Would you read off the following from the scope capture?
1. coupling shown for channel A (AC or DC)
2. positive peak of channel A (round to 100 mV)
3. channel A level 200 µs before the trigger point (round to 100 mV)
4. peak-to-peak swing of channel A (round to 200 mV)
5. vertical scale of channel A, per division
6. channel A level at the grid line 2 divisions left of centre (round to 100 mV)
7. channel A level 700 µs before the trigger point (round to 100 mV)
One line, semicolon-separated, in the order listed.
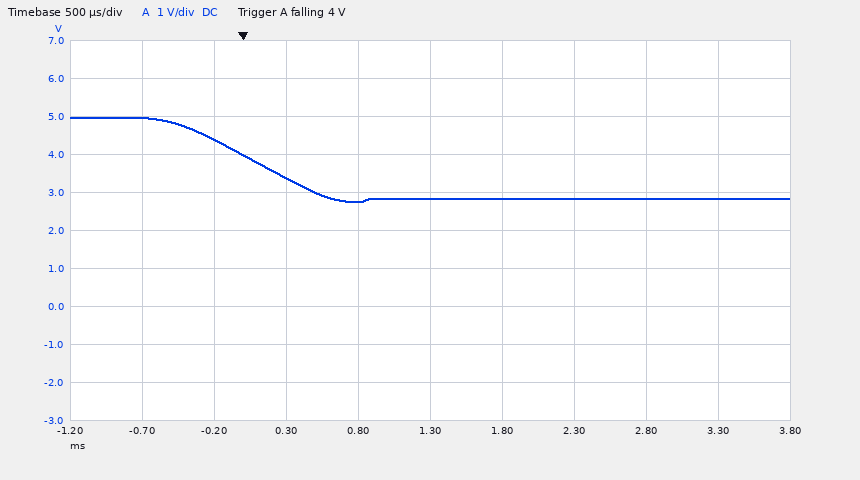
DC; 5.0 V; 4.4 V; 2.2 V; 1 V; 3.4 V; 5.0 V
